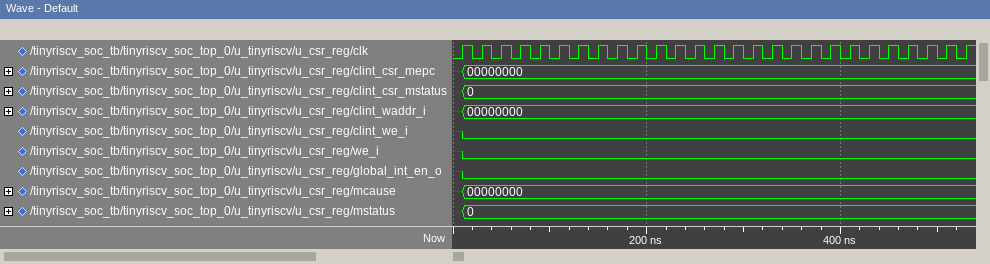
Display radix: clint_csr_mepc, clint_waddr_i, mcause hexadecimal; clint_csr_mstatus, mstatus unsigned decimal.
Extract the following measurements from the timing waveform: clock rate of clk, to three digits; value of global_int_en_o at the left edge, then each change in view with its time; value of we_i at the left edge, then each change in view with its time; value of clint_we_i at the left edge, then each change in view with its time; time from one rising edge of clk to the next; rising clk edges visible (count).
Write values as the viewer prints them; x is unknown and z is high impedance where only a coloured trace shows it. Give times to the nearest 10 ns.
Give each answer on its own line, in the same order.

50.0 MHz
x, 0 at 10 ns
x, 0 at 10 ns
x, 0 at 10 ns
20 ns
27
